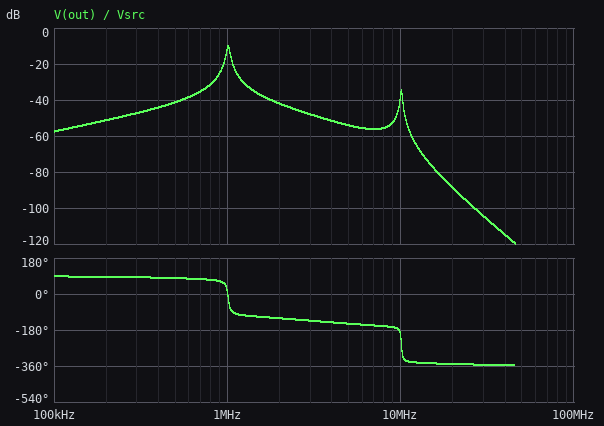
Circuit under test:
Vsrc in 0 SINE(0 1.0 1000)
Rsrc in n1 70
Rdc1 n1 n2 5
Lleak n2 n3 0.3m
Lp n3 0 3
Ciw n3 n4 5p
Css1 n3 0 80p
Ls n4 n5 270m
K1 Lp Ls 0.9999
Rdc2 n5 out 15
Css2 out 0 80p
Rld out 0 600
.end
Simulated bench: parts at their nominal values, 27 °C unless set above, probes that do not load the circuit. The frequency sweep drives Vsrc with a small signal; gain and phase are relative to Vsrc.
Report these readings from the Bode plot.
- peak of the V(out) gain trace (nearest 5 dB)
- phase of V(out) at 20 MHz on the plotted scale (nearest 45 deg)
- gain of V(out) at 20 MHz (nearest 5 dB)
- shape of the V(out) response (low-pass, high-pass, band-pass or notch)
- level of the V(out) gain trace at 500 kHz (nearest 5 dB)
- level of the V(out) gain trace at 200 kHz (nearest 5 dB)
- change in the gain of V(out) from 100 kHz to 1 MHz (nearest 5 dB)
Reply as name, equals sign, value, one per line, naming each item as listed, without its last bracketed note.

peak of the V(out) gain trace = -10 dB
phase of V(out) at 20 MHz on the plotted scale = -360 deg
gain of V(out) at 20 MHz = -90 dB
shape of the V(out) response = band-pass
level of the V(out) gain trace at 500 kHz = -40 dB
level of the V(out) gain trace at 200 kHz = -50 dB
change in the gain of V(out) from 100 kHz to 1 MHz = 45 dB
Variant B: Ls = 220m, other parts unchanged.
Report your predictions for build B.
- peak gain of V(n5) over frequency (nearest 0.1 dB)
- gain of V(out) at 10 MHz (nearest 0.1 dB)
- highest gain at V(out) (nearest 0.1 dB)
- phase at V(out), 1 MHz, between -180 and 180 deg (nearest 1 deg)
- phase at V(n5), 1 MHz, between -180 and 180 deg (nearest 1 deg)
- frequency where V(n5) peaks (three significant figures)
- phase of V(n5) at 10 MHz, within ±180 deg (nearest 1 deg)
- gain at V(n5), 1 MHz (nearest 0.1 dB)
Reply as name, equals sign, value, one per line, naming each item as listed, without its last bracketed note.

peak gain of V(n5) over frequency = -9.3 dB
gain of V(out) at 10 MHz = -53.7 dB
highest gain at V(out) = -9.5 dB
phase at V(out), 1 MHz, between -180 and 180 deg = 10 deg
phase at V(n5), 1 MHz, between -180 and 180 deg = 11 deg
frequency where V(n5) peaks = 1.01 MHz
phase of V(n5) at 10 MHz, within ±180 deg = -163 deg
gain at V(n5), 1 MHz = -10.4 dB
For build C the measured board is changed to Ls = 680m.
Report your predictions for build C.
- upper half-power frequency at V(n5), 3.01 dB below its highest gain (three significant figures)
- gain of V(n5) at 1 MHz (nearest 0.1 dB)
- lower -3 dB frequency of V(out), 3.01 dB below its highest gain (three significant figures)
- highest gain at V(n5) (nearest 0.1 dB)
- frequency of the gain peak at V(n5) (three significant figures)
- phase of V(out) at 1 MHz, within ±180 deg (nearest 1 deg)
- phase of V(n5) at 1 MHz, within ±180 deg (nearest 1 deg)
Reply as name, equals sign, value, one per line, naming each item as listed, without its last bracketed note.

upper half-power frequency at V(n5), 3.01 dB below its highest gain = 1.04 MHz
gain of V(n5) at 1 MHz = -14.5 dB
lower -3 dB frequency of V(out), 3.01 dB below its highest gain = 999 kHz
highest gain at V(n5) = -11.8 dB
frequency of the gain peak at V(n5) = 1.02 MHz
phase of V(out) at 1 MHz, within ±180 deg = 25 deg
phase of V(n5) at 1 MHz, within ±180 deg = 26 deg
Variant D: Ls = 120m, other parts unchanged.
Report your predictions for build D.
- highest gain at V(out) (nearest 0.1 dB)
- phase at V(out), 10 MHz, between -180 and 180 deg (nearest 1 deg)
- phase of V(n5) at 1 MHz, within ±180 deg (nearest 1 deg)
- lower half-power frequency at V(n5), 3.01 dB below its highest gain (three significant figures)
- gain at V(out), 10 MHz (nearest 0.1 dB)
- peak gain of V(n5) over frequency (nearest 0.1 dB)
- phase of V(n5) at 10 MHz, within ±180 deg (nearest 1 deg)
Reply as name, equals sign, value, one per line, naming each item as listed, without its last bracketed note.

highest gain at V(out) = -8.8 dB
phase at V(out), 10 MHz, between -180 and 180 deg = -164 deg
phase of V(n5) at 1 MHz, within ±180 deg = 3 deg
lower half-power frequency at V(n5), 3.01 dB below its highest gain = 987 kHz
gain at V(out), 10 MHz = -61.8 dB
peak gain of V(n5) over frequency = -8.6 dB
phase of V(n5) at 10 MHz, within ±180 deg = -159 deg
